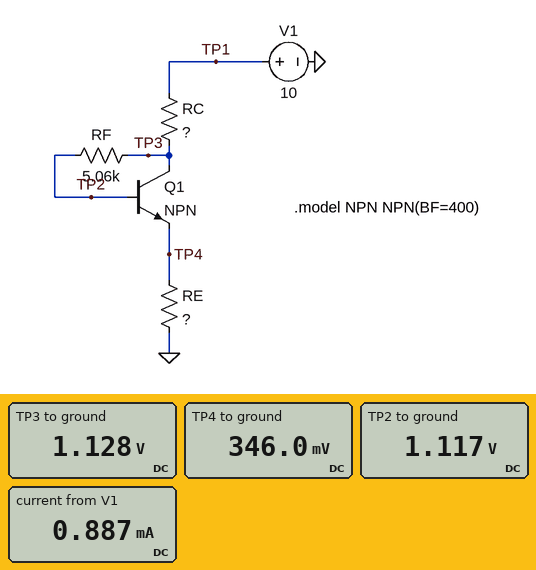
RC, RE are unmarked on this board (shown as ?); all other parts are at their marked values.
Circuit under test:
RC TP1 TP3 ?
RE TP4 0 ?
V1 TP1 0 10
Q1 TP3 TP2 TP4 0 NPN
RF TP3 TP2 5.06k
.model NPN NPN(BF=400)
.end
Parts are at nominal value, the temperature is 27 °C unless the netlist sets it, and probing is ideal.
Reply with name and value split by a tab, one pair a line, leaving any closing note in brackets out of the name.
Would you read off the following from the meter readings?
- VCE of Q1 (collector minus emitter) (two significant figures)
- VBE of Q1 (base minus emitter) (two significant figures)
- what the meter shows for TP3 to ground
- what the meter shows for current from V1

VCE of Q1 (collector minus emitter)	780 mV
VBE of Q1 (base minus emitter)	770 mV
what the meter shows for TP3 to ground	1.128 V
what the meter shows for current from V1	0.887 mA
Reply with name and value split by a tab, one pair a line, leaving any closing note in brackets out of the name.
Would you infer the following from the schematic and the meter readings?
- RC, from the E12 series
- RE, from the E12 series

RC, from the E12 series	10 kΩ
RE, from the E12 series	390 Ω
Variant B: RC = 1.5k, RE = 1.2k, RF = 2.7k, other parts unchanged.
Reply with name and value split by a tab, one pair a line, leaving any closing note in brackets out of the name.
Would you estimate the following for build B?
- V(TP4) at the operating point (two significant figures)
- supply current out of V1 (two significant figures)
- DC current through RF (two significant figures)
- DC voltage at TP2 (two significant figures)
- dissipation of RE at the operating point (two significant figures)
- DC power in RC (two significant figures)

V(TP4) at the operating point	4.1 V
supply current out of V1	3.4 mA
DC current through RF	8.5 µA
DC voltage at TP2	4.9 V
dissipation of RE at the operating point	14 mW
DC power in RC	17 mW
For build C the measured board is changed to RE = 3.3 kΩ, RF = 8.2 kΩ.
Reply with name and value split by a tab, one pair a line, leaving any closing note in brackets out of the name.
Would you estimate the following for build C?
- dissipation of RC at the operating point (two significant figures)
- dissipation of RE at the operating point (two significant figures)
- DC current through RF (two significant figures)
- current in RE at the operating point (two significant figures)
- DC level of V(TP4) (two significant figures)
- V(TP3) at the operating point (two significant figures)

dissipation of RC at the operating point	4.8 mW
dissipation of RE at the operating point	1.6 mW
DC current through RF	1.7 µA
current in RE at the operating point	690 µA
DC level of V(TP4)	2.3 V
V(TP3) at the operating point	3.1 V
